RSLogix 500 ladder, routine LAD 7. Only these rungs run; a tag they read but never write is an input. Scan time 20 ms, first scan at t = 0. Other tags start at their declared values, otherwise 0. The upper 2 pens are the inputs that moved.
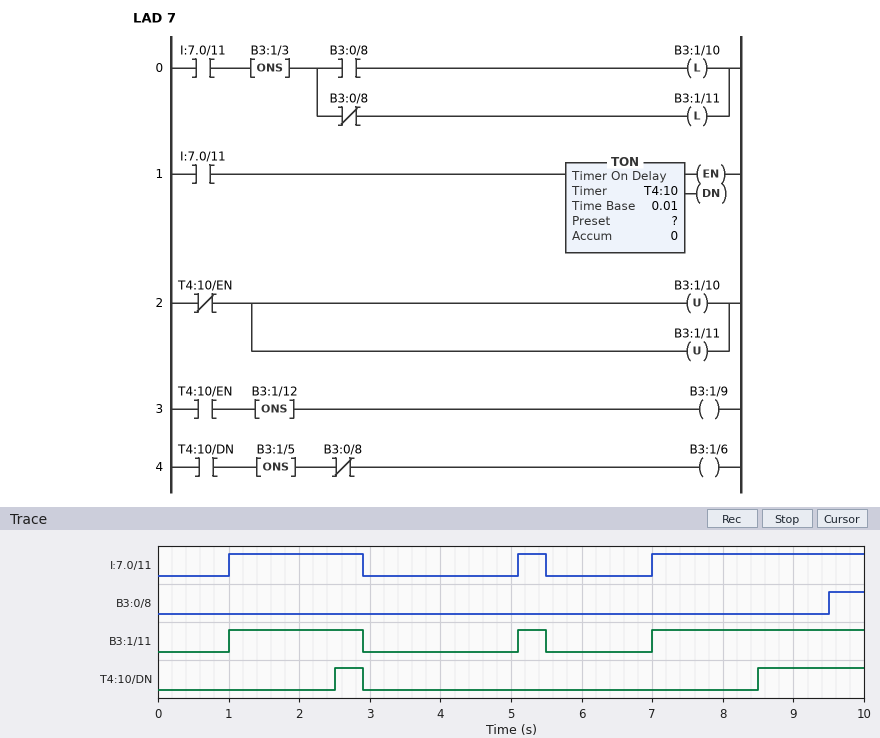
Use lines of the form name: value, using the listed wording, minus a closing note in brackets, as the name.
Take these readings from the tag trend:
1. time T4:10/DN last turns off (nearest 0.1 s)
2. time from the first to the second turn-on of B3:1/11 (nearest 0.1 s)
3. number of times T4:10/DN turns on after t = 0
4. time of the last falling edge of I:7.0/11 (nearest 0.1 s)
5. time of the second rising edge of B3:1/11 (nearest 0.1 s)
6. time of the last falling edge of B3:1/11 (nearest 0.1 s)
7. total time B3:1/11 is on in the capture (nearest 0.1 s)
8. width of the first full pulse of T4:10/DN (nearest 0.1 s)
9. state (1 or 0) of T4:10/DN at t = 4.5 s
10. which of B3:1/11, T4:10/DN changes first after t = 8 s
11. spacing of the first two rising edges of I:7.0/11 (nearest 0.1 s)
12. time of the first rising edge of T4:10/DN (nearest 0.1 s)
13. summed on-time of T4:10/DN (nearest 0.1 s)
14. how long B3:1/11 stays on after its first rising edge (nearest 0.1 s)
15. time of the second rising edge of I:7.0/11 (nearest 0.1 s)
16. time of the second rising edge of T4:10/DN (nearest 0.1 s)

time T4:10/DN last turns off: 2.9 s
time from the first to the second turn-on of B3:1/11: 4.1 s
number of times T4:10/DN turns on after t = 0: 2
time of the last falling edge of I:7.0/11: 5.5 s
time of the second rising edge of B3:1/11: 5.1 s
time of the last falling edge of B3:1/11: 5.5 s
total time B3:1/11 is on in the capture: 5.3 s
width of the first full pulse of T4:10/DN: 0.4 s
state (1 or 0) of T4:10/DN at t = 4.5 s: 0
which of B3:1/11, T4:10/DN changes first after t = 8 s: T4:10/DN
spacing of the first two rising edges of I:7.0/11: 4.1 s
time of the first rising edge of T4:10/DN: 2.5 s
summed on-time of T4:10/DN: 1.9 s
how long B3:1/11 stays on after its first rising edge: 1.9 s
time of the second rising edge of I:7.0/11: 5.1 s
time of the second rising edge of T4:10/DN: 8.5 s
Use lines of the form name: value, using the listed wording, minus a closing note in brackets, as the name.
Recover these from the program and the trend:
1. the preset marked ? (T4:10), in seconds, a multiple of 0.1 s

the preset marked ? (T4:10), in seconds, a multiple of 0.1 s: 1.5 s
